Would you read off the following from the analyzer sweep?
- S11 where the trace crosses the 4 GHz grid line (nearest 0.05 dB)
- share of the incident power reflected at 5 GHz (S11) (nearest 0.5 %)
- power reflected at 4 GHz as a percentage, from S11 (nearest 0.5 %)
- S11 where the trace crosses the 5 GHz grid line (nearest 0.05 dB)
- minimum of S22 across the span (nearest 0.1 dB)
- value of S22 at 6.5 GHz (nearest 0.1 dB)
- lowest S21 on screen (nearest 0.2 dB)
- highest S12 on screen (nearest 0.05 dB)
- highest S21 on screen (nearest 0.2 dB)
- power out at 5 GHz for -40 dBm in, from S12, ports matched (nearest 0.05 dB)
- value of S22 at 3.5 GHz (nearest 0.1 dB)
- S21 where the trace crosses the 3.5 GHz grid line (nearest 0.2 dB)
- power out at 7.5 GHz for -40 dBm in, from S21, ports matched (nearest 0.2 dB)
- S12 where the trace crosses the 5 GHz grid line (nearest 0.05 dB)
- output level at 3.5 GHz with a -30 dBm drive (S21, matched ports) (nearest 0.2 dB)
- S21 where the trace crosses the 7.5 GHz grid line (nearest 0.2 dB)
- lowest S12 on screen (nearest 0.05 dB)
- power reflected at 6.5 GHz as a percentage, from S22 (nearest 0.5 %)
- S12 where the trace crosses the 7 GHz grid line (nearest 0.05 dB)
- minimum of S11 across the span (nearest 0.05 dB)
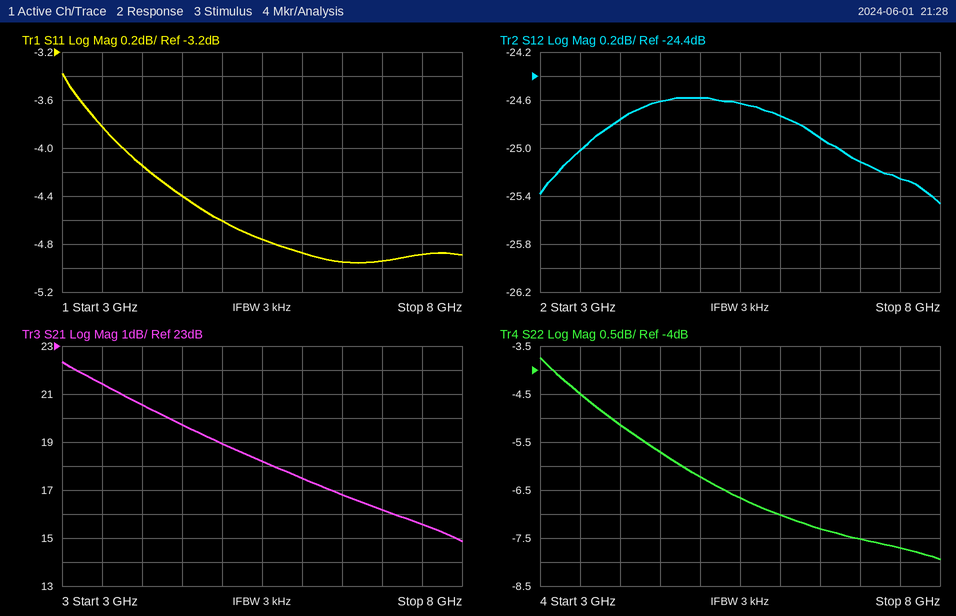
-4.15 dB
34.5 %
38.5 %
-4.60 dB
-7.9 dB
-7.3 dB
14.8 dB
-24.60 dB
22.4 dB
-64.60 dBm
-4.5 dB
21.4 dB
-24.4 dBm
-24.60 dB
-8.6 dBm
15.6 dB
-25.45 dB
18.5 %
-25.10 dB
-4.95 dB
